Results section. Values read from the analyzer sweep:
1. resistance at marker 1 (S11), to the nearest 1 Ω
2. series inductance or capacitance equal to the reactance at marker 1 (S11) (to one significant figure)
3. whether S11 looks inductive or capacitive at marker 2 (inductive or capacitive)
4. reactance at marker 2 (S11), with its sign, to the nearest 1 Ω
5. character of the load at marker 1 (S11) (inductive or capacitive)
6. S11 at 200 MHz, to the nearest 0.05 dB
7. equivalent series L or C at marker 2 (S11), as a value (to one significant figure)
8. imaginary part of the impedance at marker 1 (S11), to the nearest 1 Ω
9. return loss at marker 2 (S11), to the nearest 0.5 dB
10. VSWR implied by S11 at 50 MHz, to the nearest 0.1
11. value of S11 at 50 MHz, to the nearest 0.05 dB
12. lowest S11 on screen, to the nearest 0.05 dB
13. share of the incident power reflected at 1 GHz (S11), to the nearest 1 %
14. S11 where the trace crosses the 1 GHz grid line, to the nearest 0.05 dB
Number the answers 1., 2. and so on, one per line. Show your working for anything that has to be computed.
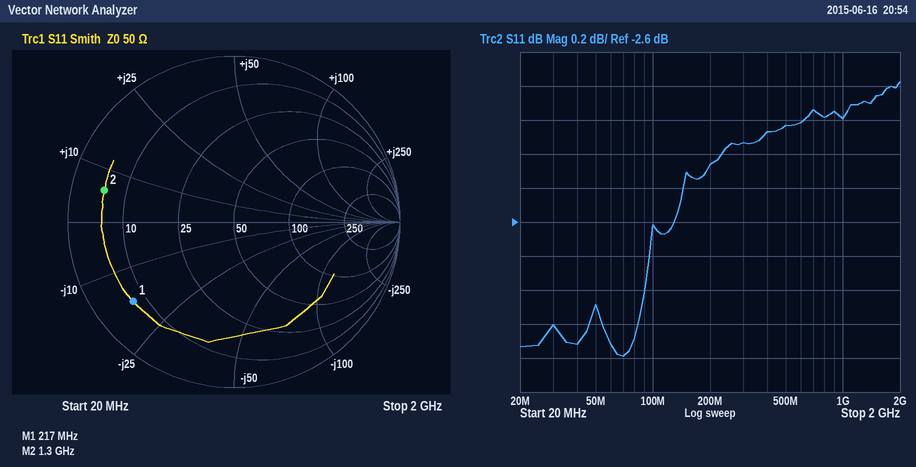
1. 7 Ω
2. C = 1/(2π × 217 MHz × 17 Ω) ≈ 43.1 pF, so 40 pF to one significant figure
3. inductive
4. +6 Ω
5. capacitive
6. -2.25 dB
7. L = 6 Ω/(2π × 1.3 GHz) ≈ 735 pH, so 700 pH to one significant figure
8. -17 Ω
9. 2.0 dB
10. |Γ| = 10^(-3.1/20) = 0.6998; VSWR = (1 + 0.6998)/(1 − 0.6998) ≈ 5.7
11. -3.10 dB
12. -3.40 dB
13. 10^(-2/10) ≈ 63 %
14. -2.00 dB
